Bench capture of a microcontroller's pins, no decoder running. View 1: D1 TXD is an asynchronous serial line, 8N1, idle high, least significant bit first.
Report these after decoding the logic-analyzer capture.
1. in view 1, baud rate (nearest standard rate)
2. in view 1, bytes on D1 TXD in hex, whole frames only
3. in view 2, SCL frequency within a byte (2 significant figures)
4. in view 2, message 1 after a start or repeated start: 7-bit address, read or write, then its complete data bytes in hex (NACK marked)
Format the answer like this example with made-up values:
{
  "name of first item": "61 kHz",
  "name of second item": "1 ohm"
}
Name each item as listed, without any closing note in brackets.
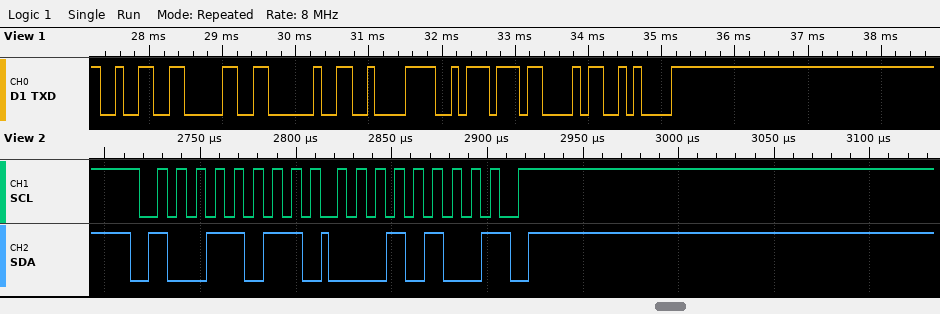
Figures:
{
  "in view 1, baud rate": "9600 baud",
  "in view 1, bytes on D1 TXD in hex, whole frames only": "32 30 20 C2 BA 43 0A",
  "in view 2, SCL frequency within a byte": "100 kHz",
  "in view 2, message 1 after a start or repeated start: 7-bit address, read or write, then its complete data bytes in hex": "0x4D read: 14 NACK"
}
